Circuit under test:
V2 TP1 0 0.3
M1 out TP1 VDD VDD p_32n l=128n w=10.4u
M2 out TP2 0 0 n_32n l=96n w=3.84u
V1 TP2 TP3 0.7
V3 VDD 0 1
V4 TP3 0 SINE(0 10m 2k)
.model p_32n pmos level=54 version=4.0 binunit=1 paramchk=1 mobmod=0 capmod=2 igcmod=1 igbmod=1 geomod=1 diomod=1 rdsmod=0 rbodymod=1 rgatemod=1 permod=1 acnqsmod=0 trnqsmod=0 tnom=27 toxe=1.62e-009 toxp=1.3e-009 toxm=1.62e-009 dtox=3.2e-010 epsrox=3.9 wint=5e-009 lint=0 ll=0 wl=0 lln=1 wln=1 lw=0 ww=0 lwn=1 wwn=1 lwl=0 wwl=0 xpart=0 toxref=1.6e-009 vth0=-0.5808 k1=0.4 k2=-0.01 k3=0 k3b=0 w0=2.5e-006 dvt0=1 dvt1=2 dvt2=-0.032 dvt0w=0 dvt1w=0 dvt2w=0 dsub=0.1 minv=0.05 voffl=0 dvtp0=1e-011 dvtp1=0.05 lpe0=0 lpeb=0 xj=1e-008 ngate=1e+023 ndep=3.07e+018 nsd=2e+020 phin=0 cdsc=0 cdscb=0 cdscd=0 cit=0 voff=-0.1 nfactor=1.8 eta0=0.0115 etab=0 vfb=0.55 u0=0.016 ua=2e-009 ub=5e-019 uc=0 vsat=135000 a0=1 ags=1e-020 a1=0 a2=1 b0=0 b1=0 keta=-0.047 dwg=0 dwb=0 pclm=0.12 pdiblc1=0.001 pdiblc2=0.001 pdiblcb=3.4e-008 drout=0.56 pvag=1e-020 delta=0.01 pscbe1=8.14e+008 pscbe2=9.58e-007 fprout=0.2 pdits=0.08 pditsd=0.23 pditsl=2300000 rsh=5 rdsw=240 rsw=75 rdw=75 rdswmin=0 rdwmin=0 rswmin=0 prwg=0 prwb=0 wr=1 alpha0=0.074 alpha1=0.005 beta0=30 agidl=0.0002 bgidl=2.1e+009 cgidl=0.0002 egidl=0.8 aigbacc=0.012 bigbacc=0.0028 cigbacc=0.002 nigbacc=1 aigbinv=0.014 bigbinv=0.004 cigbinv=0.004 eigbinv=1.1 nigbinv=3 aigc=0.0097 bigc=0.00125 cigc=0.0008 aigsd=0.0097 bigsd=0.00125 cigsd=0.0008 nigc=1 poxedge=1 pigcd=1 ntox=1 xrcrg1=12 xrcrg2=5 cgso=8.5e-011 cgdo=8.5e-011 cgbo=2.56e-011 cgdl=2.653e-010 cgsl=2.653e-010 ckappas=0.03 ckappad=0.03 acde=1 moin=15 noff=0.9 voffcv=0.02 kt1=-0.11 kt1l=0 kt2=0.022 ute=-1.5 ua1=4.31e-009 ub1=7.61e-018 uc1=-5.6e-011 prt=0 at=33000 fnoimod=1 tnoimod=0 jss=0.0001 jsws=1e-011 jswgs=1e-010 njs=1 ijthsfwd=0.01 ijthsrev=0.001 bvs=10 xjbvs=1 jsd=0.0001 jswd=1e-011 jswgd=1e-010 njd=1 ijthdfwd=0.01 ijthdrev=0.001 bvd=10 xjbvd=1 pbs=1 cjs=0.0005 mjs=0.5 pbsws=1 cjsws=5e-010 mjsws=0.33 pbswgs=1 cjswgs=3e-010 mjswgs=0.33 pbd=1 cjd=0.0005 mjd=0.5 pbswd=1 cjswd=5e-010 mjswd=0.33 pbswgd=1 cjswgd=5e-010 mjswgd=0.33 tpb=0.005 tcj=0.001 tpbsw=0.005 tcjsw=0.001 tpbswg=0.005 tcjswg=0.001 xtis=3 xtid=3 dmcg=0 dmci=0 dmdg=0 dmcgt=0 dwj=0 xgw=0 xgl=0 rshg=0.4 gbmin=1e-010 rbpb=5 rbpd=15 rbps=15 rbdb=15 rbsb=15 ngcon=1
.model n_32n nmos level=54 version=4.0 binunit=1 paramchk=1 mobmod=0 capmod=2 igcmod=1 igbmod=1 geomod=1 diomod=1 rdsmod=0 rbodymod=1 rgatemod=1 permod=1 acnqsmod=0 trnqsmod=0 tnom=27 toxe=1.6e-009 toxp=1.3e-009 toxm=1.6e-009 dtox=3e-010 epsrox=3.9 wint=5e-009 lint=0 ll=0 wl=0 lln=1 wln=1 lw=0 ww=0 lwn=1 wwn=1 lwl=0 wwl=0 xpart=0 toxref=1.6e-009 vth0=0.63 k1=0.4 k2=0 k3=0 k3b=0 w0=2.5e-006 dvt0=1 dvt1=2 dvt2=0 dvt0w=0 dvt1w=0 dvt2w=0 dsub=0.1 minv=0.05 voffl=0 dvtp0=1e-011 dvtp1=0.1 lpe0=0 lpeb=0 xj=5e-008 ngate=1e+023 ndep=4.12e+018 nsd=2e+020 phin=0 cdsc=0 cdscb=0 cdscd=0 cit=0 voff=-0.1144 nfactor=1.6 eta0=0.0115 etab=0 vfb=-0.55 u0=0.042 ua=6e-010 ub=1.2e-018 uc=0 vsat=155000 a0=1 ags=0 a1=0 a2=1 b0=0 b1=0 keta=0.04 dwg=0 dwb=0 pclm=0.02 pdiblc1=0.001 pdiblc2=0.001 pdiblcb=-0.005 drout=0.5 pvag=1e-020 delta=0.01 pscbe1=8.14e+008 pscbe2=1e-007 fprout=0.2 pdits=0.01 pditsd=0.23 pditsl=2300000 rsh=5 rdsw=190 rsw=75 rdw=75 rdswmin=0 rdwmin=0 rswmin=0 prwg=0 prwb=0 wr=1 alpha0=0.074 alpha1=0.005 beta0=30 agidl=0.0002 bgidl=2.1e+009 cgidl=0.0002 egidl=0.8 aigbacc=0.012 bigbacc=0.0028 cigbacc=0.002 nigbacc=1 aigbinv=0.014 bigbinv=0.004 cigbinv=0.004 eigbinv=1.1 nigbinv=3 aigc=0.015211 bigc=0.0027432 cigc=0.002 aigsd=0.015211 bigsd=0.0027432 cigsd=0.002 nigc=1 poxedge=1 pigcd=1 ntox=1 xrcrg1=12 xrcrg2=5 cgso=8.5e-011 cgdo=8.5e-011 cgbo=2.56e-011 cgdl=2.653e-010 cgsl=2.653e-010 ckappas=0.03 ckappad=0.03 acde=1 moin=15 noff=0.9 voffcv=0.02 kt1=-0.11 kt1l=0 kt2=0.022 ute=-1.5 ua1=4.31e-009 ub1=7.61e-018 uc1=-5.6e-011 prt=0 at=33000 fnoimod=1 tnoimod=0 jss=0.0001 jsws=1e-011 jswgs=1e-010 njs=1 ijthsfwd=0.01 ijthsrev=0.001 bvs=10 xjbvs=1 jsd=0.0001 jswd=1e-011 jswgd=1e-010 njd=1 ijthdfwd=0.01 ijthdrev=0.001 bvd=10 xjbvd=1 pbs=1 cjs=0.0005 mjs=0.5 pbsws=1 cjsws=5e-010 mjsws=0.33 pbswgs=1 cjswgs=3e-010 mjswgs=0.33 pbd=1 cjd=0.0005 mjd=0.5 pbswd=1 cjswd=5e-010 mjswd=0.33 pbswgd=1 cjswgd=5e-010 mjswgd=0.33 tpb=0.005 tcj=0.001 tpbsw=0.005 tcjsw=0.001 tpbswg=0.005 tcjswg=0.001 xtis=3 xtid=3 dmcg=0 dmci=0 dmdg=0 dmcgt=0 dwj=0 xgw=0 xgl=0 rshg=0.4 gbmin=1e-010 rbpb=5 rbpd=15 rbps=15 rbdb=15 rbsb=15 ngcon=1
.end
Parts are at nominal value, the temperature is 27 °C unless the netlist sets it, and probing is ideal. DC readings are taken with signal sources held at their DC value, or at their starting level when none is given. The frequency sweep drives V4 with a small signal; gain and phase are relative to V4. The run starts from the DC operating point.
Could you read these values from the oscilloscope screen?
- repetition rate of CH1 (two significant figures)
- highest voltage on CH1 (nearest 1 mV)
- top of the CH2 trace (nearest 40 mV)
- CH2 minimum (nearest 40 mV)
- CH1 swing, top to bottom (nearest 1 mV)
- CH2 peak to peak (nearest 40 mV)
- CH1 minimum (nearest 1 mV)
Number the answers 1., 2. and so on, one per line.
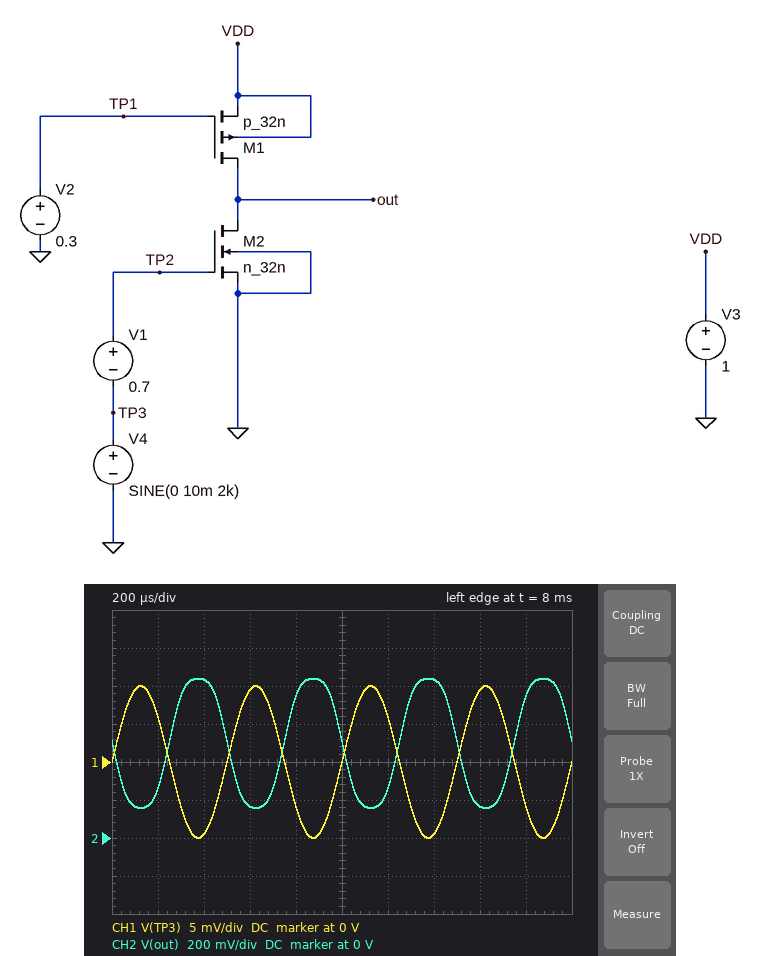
1. 2.0 kHz
2. 10 mV
3. 840 mV
4. 160 mV
5. 20 mV
6. 680 mV
7. -10 mV
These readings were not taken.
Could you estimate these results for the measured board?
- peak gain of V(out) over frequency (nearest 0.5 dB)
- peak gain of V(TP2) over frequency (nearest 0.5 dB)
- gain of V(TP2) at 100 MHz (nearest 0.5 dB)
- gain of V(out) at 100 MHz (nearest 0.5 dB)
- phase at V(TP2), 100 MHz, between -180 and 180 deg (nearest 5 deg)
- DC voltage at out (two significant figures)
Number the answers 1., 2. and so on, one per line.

1. 33.0 dB
2. 0 dB
3. 0 dB
4. 32.5 dB
5. 0 deg
6. 510 mV
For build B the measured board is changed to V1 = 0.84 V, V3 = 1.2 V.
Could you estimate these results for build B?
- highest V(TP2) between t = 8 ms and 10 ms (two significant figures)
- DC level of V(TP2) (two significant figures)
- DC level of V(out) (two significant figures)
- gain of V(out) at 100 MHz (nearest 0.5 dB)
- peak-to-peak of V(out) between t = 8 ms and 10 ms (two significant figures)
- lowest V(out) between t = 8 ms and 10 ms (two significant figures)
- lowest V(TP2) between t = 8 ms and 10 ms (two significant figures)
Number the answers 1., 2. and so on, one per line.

1. 850 mV
2. 840 mV
3. 1.0 V
4. 8.0 dB
5. 51 mV
6. 970 mV
7. 830 mV
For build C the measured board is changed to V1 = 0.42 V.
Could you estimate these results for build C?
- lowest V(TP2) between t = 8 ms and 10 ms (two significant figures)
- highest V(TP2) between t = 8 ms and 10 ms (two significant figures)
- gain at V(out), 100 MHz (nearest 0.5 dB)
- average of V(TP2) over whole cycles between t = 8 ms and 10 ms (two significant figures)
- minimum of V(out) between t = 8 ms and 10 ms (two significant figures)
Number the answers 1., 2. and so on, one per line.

1. 410 mV
2. 430 mV
3. -43.0 dB
4. 420 mV
5. 1.0 V
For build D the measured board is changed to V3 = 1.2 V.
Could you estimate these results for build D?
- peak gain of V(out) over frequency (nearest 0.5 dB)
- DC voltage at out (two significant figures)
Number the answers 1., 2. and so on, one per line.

1. -5.5 dB
2. 1.2 V
